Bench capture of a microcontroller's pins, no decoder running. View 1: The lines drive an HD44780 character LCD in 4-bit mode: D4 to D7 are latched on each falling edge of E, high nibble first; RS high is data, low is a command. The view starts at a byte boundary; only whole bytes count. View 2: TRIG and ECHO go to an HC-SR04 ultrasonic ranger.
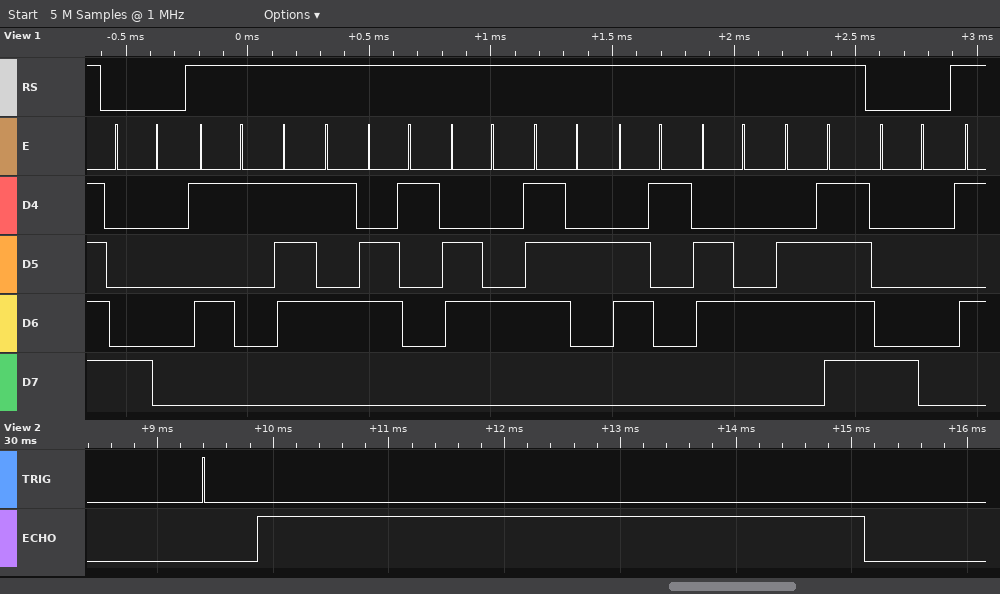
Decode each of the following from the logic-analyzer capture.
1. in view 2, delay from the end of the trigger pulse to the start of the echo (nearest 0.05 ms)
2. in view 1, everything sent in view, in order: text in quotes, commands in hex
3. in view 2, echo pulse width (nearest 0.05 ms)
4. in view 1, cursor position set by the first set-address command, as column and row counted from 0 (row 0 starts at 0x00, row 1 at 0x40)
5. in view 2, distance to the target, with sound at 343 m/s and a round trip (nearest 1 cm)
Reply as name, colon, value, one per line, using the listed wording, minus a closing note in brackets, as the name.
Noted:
in view 2, delay from the end of the trigger pulse to the start of the echo: 0.45 ms
in view 1, everything sent in view, in order: text in quotes, commands in hex: 0x80 "Quadrado" 0x80
in view 2, echo pulse width: 5.25 ms
in view 1, cursor position set by the first set-address command, as column and row counted from 0: column 0, row 0
in view 2, distance to the target, with sound at 343 m/s and a round trip: 90 cm
